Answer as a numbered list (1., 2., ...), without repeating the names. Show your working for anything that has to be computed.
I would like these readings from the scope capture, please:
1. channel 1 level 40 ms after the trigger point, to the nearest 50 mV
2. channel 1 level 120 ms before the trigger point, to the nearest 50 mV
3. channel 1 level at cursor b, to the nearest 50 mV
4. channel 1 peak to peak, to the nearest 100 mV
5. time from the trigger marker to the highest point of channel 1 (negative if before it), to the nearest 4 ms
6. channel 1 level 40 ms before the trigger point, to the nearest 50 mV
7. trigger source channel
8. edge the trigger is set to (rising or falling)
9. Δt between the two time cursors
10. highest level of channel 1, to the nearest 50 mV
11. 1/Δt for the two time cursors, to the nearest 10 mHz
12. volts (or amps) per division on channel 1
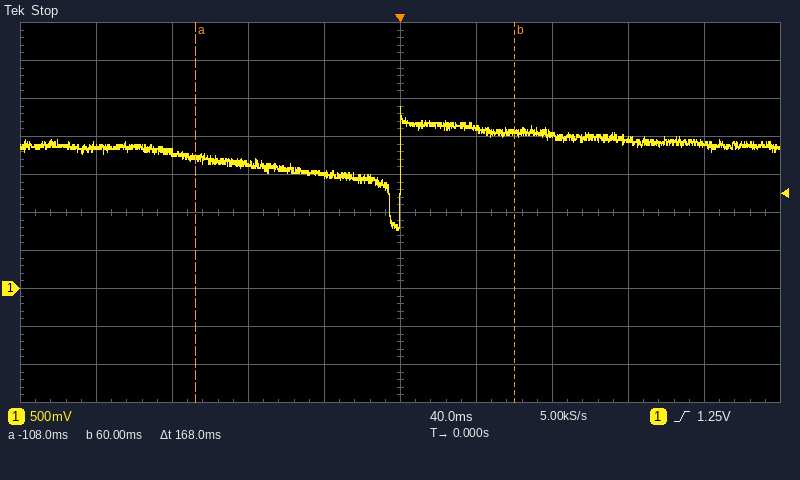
1. 2.10 V
2. 1.80 V
3. 2.05 V
4. 1.60 V
5. 0 ms
6. 1.50 V
7. channel 1
8. rising
9. 168 ms
10. 2.40 V
11. 1 / 168 ms ≈ 5.95 Hz
12. 500 mV
